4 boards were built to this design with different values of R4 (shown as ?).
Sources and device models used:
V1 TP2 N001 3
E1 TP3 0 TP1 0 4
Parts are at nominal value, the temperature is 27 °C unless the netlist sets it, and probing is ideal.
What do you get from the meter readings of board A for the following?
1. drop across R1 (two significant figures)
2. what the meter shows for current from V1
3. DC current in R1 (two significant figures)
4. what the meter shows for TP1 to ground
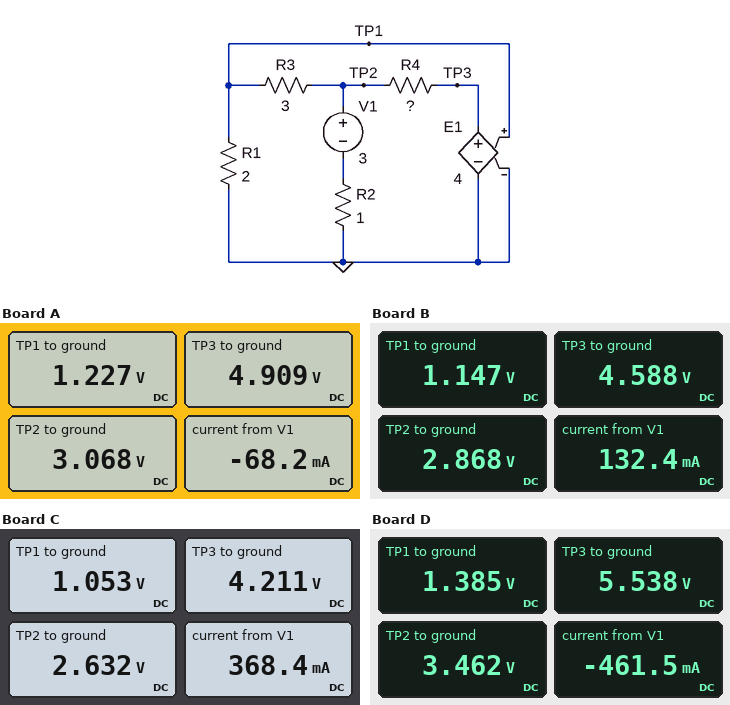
1.2 V
-68.2 mA
610 mA
1.227 V
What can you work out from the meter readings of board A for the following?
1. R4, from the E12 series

2.7 Ω
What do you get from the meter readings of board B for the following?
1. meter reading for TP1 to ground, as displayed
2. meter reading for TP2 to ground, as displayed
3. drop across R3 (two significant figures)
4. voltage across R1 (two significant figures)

1.147 V
2.868 V
1.7 V
1.1 V
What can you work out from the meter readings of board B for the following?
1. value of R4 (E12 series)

3.9 Ω
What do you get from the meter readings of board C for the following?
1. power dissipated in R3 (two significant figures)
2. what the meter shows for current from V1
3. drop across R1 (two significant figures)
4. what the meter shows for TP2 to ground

830 mW
368.4 mA
1.1 V
2.632 V
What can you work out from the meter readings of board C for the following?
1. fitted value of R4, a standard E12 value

10 Ω
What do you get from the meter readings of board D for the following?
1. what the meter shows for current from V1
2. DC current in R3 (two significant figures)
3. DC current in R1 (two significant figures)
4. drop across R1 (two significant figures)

-461.5 mA
690 mA
690 mA
1.4 V
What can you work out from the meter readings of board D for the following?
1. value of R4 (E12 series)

1.8 Ω
